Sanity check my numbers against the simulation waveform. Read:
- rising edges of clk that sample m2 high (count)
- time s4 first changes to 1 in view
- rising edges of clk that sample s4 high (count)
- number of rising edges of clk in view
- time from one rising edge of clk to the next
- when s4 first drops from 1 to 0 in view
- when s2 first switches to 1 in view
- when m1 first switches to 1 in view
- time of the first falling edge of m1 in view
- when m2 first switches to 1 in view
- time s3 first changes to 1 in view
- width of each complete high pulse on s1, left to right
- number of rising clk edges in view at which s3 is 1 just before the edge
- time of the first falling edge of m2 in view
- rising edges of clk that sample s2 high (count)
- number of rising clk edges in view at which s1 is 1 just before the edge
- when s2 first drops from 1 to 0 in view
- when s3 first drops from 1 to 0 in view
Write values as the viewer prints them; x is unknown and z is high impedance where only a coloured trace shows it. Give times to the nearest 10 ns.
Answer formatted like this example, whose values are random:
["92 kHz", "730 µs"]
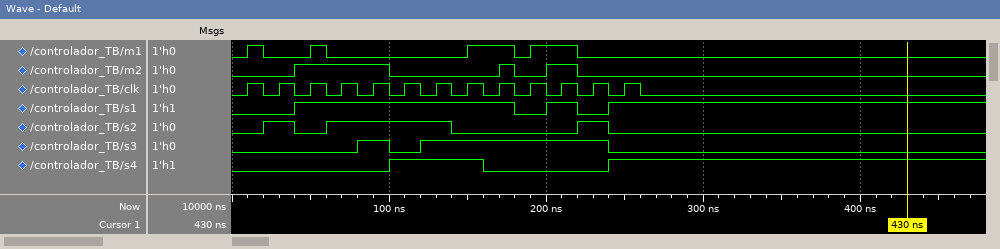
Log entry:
["4", "100 ns", "4", "13", "20 ns", "160 ns", "20 ns", "10 ns", "20 ns", "40 ns", "80 ns", "140 ns, 20 ns", "7", "100 ns", "6", "9", "40 ns", "100 ns"]
